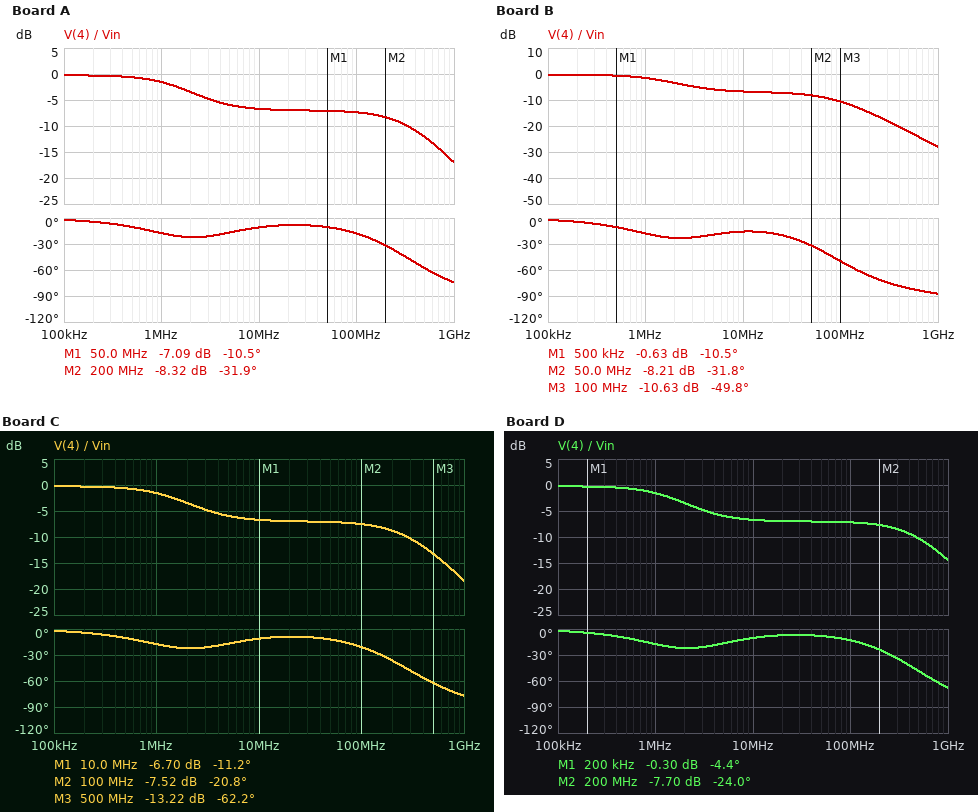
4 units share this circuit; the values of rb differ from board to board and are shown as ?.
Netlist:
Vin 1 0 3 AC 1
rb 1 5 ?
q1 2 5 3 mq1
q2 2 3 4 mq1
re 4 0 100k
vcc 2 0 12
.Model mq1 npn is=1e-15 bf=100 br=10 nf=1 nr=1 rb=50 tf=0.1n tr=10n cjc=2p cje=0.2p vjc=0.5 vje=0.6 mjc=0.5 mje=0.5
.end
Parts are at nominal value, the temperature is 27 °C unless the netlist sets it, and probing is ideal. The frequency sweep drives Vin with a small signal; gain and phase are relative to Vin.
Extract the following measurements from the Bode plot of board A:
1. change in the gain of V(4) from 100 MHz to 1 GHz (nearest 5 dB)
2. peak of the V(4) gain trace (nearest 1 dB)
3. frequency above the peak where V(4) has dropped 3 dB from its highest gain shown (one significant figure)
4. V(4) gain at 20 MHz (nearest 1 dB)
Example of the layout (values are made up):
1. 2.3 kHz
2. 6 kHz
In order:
1. -10 dB
2. 0 dB
3. 2 MHz
4. -7 dB
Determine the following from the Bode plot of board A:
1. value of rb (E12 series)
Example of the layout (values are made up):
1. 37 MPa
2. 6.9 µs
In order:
1. 680 Ω
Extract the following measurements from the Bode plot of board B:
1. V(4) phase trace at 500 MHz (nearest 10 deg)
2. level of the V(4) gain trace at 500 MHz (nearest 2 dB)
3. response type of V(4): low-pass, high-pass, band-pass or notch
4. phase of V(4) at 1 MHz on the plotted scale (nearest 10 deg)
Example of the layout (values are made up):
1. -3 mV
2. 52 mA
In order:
1. -80 deg
2. -22 dB
3. low-pass
4. -20 deg
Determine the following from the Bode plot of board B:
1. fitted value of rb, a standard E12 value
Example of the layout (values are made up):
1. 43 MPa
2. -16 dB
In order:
1. 2.7 kΩ
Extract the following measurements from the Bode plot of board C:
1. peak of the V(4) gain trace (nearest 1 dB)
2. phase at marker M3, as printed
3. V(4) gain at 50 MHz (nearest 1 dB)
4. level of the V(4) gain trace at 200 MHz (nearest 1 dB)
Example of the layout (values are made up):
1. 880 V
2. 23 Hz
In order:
1. 0 dB
2. -62.2 deg
3. -7 dB
4. -9 dB
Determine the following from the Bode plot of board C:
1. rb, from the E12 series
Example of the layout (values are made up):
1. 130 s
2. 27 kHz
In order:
1. 820 Ω
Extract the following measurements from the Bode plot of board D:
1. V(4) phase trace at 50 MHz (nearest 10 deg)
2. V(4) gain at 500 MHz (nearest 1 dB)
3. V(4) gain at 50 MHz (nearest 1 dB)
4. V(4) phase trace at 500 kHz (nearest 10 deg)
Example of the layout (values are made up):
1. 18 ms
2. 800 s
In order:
1. -10 deg
2. -10 dB
3. -7 dB
4. -10 deg
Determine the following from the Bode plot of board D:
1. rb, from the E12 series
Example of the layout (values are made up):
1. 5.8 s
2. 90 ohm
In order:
1. 470 Ω
